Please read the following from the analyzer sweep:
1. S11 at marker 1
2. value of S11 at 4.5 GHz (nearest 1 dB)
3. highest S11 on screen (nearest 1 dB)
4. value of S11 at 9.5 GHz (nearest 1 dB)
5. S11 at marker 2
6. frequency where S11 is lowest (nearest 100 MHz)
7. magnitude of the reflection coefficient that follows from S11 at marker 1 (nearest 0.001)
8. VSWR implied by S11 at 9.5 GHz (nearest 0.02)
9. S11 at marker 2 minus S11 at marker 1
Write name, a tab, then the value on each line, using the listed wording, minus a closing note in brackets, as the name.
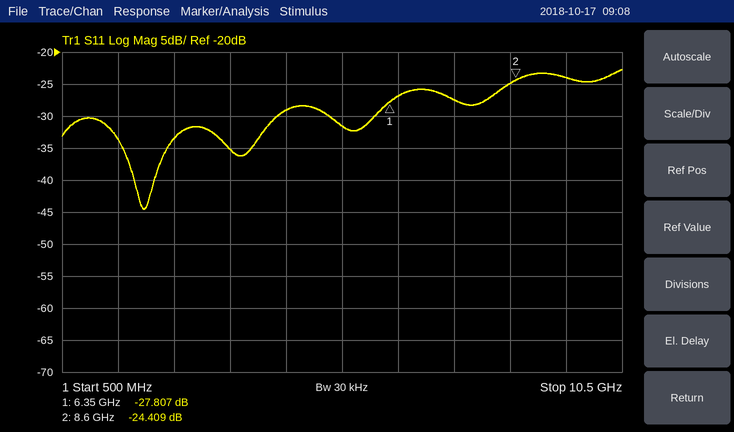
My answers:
S11 at marker 1	-27.807 dB
value of S11 at 4.5 GHz	-29 dB
highest S11 on screen	-23 dB
value of S11 at 9.5 GHz	-24 dB
S11 at marker 2	-24.409 dB
frequency where S11 is lowest	2.0 GHz
magnitude of the reflection coefficient that follows from S11 at marker 1	0.041
VSWR implied by S11 at 9.5 GHz	1.14
S11 at marker 2 minus S11 at marker 1	3.398 dB
